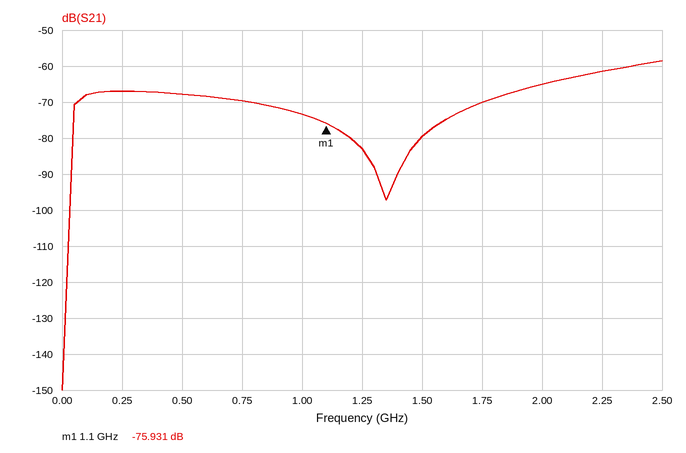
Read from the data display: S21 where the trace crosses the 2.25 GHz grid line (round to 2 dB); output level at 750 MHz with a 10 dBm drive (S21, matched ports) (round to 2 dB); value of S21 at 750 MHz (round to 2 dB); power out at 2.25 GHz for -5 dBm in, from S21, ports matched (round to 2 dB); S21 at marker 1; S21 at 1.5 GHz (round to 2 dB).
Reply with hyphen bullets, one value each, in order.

- -62 dB
- -60 dBm
- -70 dB
- -66 dBm
- -75.931 dB
- -80 dB
